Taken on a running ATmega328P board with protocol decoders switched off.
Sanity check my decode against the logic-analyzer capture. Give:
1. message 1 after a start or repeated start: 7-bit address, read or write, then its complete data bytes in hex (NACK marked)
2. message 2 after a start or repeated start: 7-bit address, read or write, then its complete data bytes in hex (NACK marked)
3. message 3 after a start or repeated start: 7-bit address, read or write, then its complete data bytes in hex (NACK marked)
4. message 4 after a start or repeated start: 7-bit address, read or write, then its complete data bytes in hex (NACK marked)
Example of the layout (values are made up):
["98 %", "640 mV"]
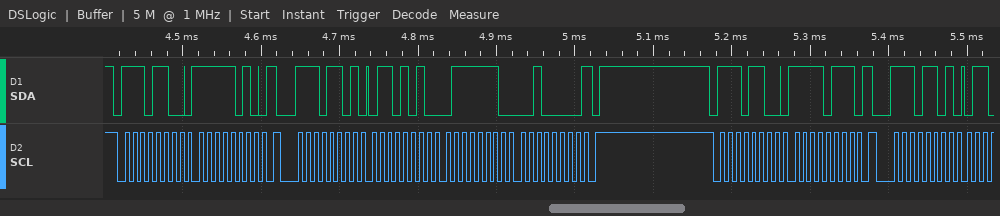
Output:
["0x76 write: FA", "0x76 read: 6A 7E 20 NACK", "0x76 write: F7", "0x76 read"]
